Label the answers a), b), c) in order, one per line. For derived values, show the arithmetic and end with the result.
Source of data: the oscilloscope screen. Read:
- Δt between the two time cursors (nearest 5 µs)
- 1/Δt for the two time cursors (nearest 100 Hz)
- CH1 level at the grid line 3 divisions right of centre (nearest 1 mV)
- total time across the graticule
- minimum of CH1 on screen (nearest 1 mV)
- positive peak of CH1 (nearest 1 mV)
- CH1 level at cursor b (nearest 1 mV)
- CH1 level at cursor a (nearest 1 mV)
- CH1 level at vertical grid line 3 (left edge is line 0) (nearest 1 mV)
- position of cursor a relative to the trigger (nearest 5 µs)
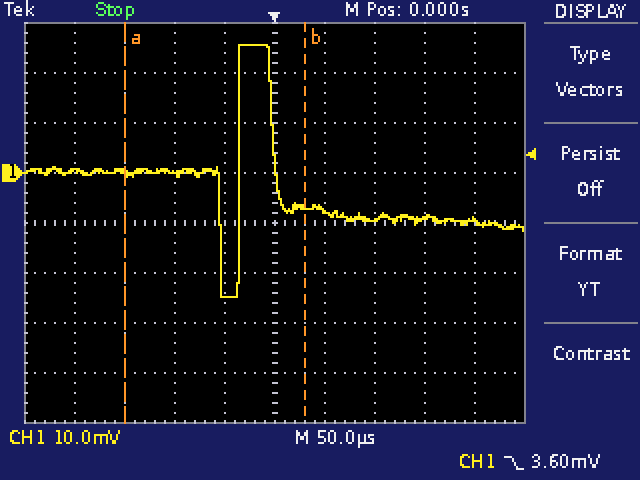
a) 180 µs
b) 1 / 180 µs ≈ 5.6 kHz
c) -9 mV
d) 500 µs
e) -25 mV
f) 26 mV
g) -7 mV
h) 0 mV
i) 0 mV
j) -150 µs
